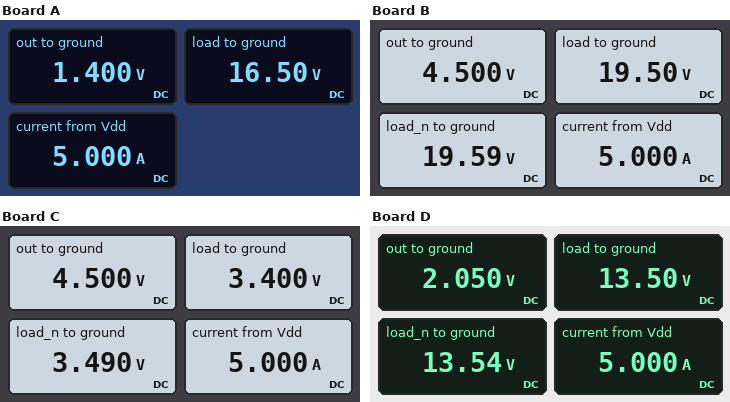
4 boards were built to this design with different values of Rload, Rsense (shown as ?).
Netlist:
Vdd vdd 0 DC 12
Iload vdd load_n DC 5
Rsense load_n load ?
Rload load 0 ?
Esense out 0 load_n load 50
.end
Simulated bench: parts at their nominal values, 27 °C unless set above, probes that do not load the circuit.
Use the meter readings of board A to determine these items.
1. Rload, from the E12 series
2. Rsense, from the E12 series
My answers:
3.3 Ω
5.6 mΩ
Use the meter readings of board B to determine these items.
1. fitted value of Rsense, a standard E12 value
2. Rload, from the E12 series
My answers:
0.018 Ω
3.9 Ω
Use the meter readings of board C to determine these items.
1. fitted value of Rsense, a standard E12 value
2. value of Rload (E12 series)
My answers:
0.018 Ω
0.68 Ω
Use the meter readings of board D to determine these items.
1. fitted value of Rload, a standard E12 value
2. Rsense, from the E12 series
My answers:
2.7 Ω
8.2 mΩ
